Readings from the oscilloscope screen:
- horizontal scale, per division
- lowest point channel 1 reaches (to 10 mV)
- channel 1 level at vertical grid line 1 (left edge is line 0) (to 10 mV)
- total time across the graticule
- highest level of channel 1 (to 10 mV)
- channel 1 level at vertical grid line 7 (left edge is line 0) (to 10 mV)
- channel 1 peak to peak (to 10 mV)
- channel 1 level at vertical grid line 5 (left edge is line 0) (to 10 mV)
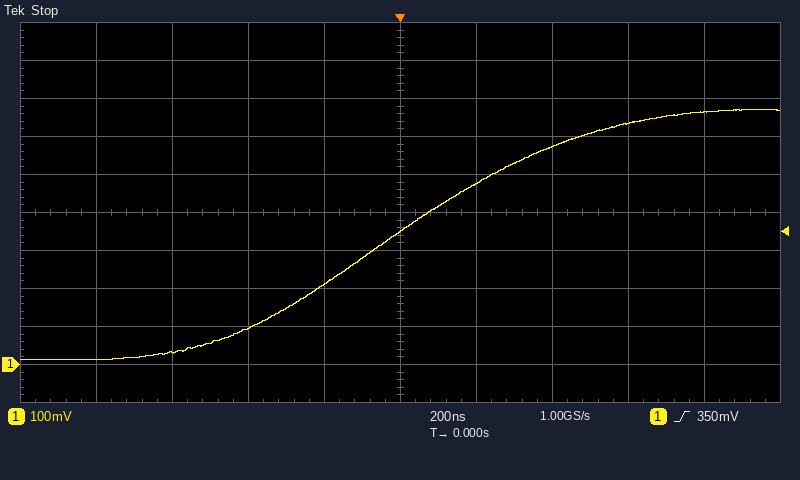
200 ns
10 mV
10 mV
2 µs
670 mV
570 mV
660 mV
350 mV
